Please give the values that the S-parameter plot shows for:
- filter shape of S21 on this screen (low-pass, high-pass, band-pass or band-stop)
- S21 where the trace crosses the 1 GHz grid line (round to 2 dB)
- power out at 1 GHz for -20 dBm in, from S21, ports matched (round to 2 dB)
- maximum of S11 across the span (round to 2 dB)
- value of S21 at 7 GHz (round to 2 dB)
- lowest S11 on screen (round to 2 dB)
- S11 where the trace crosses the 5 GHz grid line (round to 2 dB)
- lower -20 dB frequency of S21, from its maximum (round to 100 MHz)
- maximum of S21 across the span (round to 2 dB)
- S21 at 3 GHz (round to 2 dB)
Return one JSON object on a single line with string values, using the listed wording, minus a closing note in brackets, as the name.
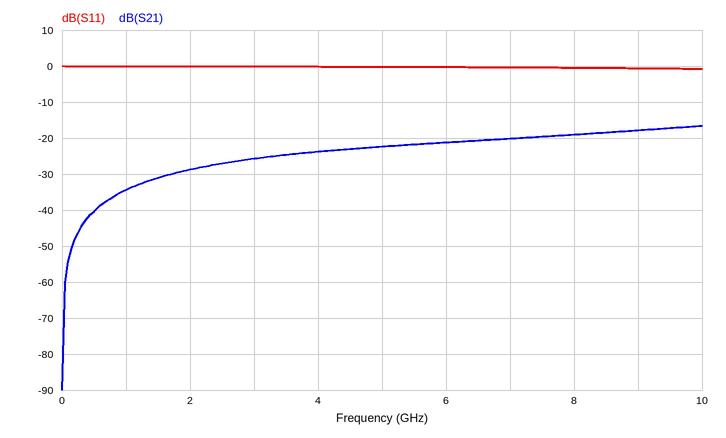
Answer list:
{"filter shape of S21 on this screen": "high-pass", "S21 where the trace crosses the 1 GHz grid line": "-34 dB", "power out at 1 GHz for -20 dBm in, from S21, ports matched": "-54 dBm", "maximum of S11 across the span": "0 dB", "value of S21 at 7 GHz": "-20 dB", "lowest S11 on screen": "0 dB", "S11 where the trace crosses the 5 GHz grid line": "0 dB", "lower -20 dB frequency of S21, from its maximum": "800 MHz", "maximum of S21 across the span": "-16 dB", "S21 at 3 GHz": "-26 dB"}
